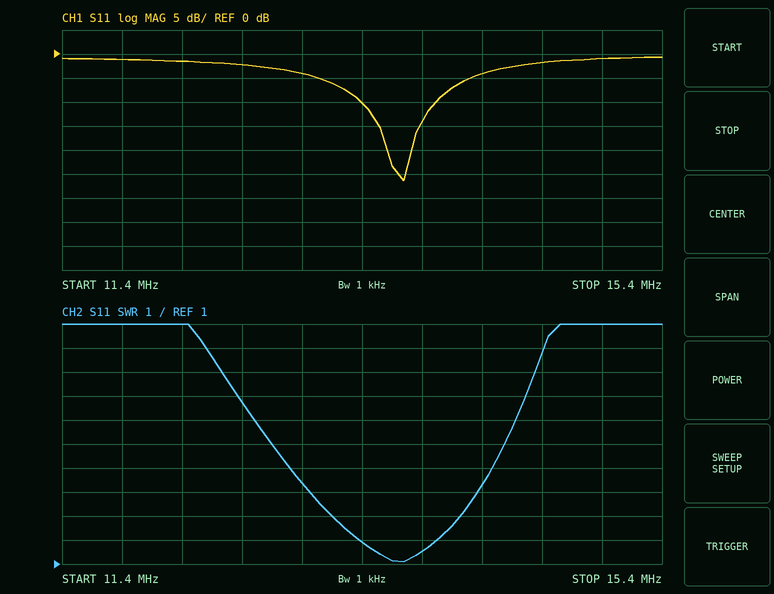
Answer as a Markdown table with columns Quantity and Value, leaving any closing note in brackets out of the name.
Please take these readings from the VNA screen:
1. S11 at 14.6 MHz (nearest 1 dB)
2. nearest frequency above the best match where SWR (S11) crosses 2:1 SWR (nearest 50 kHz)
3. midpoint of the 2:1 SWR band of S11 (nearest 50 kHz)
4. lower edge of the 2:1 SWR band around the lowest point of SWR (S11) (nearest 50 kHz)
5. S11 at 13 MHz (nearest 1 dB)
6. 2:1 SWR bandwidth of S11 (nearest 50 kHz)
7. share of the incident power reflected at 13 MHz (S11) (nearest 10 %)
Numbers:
| Quantity | Value |
|---|---|
| S11 at 14.6 MHz | -2 dB |
| nearest frequency above the best match where SWR (S11) crosses 2:1 SWR | 13.90 MHz |
| midpoint of the 2:1 SWR band of S11 | 13.65 MHz |
| lower edge of the 2:1 SWR band around the lowest point of SWR (S11) | 13.40 MHz |
| S11 at 13 MHz | -4 dB |
| 2:1 SWR bandwidth of S11 | 500 kHz |
| share of the incident power reflected at 13 MHz (S11) | 40 % |
